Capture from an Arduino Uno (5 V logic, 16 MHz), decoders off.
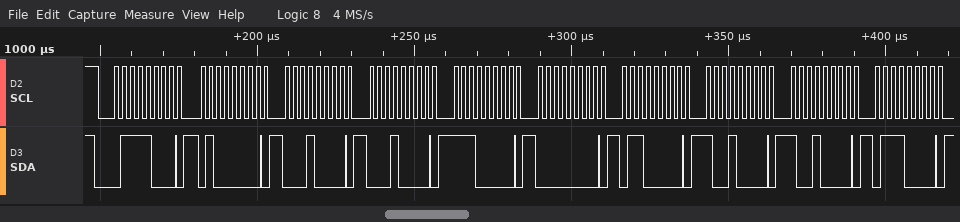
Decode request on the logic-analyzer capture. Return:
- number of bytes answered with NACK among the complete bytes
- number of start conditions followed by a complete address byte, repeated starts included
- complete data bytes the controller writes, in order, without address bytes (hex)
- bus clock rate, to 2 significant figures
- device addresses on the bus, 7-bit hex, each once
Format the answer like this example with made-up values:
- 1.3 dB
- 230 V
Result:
- 0
- 1
- 40 10 10 E0 00 60 90 90 70
- 400 kHz
- 0x3C
